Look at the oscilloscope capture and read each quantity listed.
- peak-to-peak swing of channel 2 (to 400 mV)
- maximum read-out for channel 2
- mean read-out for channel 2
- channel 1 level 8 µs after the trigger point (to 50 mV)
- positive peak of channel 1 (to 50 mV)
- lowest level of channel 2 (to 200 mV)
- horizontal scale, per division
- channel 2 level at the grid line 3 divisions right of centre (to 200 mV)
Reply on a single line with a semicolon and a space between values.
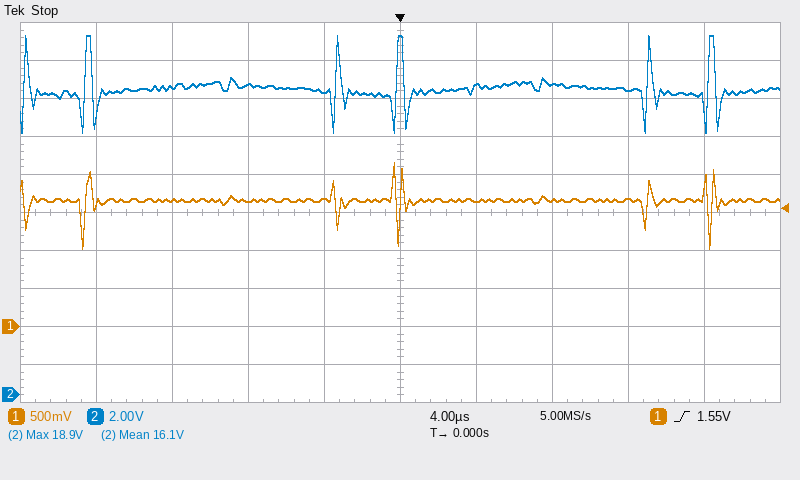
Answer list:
5.2 V; 18.9 V; 16.1 V; 1.65 V; 2.15 V; 13.8 V; 4 µs; 16.0 V
